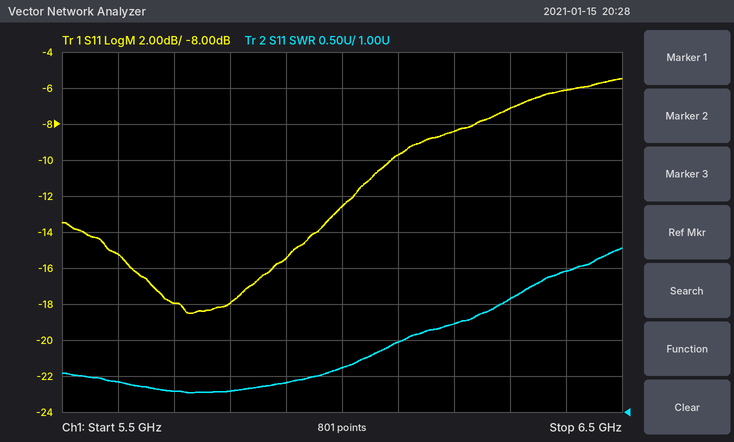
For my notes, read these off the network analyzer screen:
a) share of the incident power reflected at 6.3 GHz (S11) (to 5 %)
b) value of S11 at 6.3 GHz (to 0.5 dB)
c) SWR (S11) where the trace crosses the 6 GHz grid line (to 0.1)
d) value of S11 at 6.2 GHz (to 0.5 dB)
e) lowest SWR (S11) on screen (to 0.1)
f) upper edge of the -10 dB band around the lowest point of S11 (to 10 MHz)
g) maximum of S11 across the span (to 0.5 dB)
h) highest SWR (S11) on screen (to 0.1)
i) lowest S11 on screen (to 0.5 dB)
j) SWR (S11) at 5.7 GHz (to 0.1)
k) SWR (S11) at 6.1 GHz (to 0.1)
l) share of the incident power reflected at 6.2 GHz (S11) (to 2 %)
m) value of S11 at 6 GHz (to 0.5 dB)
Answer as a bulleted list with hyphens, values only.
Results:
- 20 %
- -7.0 dB
- 1.6
- -8.5 dB
- 1.3
- 6.09 GHz
- -5.5 dB
- 3.3
- -18.5 dB
- 1.3
- 2.0
- 14 %
- -12.5 dB
